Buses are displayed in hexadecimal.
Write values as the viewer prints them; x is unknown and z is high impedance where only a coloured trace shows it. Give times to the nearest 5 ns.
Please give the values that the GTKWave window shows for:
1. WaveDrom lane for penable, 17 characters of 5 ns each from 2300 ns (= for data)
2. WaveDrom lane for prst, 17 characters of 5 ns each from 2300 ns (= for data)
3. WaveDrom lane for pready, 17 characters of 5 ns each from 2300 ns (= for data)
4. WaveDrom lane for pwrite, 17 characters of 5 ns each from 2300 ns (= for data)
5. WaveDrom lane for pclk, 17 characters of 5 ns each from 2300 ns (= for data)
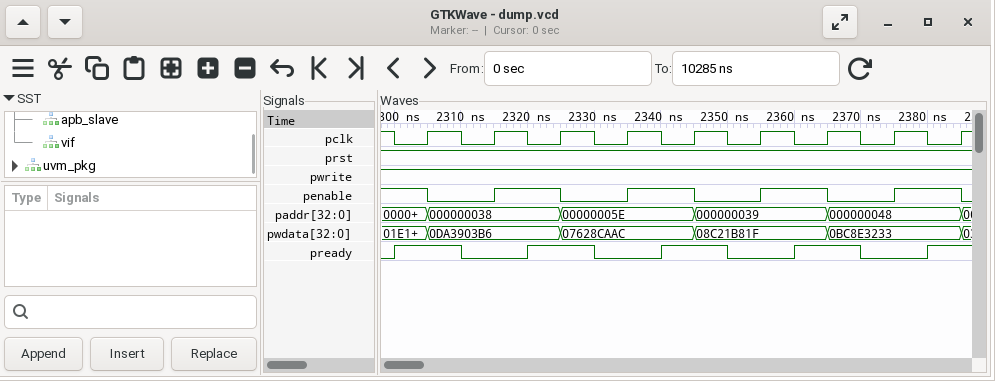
{name: 'penable', wave: '10.1.0.1.0.1.0.1.'}
{name: 'prst', wave: '1................'}
{name: 'pready', wave: '1.0.1.0.1.0.1.0.1'}
{name: 'pwrite', wave: '1................'}
{name: 'pclk', wave: '01010101010101010'}
